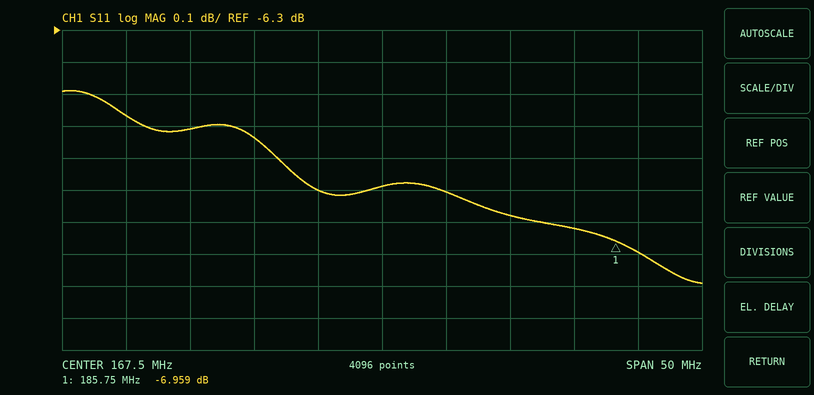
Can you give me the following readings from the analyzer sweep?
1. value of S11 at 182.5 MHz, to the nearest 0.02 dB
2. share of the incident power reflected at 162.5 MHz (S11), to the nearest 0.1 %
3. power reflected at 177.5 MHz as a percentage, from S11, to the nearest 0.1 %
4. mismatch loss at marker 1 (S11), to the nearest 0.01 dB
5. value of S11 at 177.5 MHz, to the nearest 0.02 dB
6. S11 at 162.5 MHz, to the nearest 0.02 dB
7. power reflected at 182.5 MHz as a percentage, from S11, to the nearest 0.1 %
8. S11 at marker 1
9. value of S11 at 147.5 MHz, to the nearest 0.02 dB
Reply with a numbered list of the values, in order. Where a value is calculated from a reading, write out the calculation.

1. -6.92 dB
2. 10^(-6.8/10) ≈ 20.9 %
3. 10^(-6.88/10) ≈ 20.5 %
4. −10 log10(1 − 10^(-6.959/10)) ≈ 0.98 dB
5. -6.88 dB
6. -6.80 dB
7. 10^(-6.92/10) ≈ 20.3 %
8. -6.959 dB
9. -6.56 dB
